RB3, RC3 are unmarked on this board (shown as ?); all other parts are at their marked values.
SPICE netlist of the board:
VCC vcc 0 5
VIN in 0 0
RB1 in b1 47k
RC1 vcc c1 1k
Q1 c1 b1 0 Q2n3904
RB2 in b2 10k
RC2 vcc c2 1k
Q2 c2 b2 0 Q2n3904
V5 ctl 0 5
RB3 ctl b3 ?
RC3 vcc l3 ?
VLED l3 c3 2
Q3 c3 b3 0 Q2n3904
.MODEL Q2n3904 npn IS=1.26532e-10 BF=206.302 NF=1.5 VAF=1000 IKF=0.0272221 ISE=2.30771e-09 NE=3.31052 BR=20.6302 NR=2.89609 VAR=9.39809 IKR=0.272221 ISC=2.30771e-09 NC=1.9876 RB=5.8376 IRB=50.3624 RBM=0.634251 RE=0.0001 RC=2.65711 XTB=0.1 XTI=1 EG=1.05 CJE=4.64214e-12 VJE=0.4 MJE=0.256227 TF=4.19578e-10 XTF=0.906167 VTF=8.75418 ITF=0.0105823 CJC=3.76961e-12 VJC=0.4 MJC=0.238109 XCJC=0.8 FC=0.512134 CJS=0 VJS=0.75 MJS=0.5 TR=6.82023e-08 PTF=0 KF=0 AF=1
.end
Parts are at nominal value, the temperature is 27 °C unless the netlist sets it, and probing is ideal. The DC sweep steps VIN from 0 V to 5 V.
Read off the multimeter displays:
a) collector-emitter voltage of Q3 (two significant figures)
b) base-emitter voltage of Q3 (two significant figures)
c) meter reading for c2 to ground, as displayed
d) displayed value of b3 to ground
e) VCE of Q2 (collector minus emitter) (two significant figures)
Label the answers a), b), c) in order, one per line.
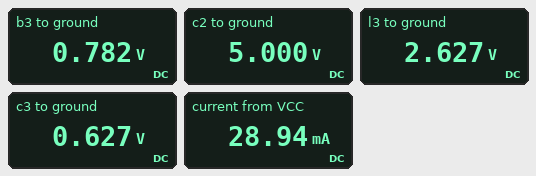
a) 630 mV
b) 780 mV
c) 5.000 V
d) 0.782 V
e) 5.0 V
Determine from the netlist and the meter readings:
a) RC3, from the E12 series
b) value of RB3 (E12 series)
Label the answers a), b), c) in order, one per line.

a) 82 Ω
b) 12 kΩ
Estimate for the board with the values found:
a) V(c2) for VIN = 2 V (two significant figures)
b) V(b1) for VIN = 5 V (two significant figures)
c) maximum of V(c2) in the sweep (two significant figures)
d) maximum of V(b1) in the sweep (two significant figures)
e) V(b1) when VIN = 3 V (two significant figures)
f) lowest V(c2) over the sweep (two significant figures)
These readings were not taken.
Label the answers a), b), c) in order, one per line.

a) 160 mV
b) 690 mV
c) 5.0 V
d) 690 mV
e) 690 mV
f) 86 mV
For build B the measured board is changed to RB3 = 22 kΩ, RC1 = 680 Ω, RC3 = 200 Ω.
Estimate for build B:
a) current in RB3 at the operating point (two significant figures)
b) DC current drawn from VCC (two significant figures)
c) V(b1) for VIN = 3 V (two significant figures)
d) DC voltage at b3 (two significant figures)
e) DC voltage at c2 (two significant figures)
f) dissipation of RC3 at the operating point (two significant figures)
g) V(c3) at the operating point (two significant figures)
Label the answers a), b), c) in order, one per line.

a) 190 µA
b) 14 mA
c) 700 mV
d) 740 mV
e) 5.0 V
f) 38 mW
g) 250 mV
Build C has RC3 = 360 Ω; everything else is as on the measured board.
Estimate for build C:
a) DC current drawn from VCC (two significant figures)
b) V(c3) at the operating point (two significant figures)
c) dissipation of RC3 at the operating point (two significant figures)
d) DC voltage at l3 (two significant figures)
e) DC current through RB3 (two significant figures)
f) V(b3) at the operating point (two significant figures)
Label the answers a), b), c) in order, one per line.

a) 8.0 mA
b) 130 mV
c) 23 mW
d) 2.1 V
e) 360 µA
f) 710 mV
